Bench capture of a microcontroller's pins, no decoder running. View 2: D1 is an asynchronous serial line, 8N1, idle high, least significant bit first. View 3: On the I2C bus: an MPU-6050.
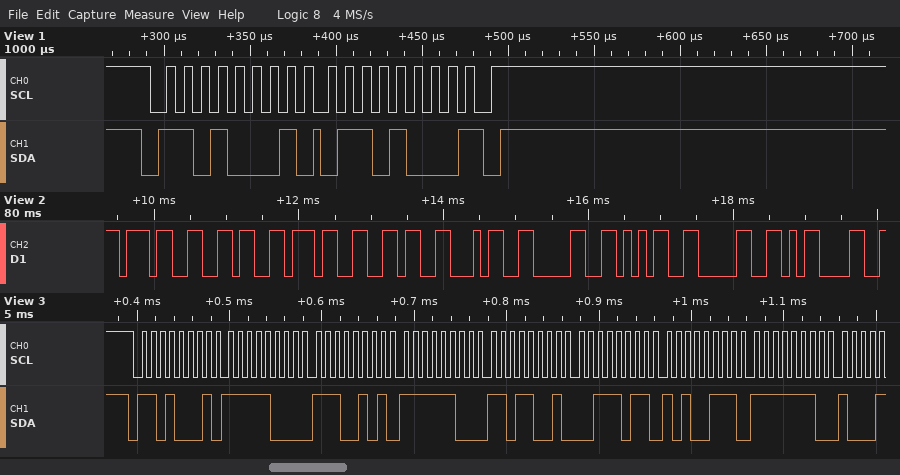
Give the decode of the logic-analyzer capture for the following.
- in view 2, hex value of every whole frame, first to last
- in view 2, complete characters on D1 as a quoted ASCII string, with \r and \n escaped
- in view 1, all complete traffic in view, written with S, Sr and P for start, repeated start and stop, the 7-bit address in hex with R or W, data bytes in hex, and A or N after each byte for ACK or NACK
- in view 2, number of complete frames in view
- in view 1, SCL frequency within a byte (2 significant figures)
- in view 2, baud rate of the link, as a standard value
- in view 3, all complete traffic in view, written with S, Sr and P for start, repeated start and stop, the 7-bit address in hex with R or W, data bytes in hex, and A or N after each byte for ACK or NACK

37 36 37 36 34 30 35 30 0D
"76764050\r"
S 68R A 68 N P
9
100 kHz
9600 baud
S 68R A F8 A E5 A FC A D9 A 3B A A7 A FE A
